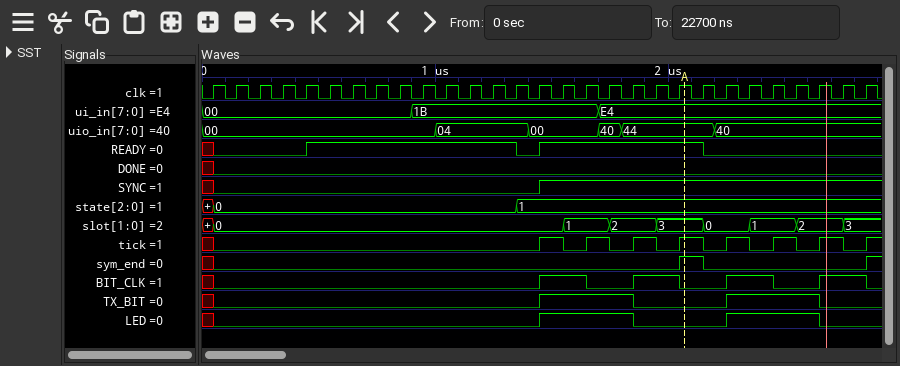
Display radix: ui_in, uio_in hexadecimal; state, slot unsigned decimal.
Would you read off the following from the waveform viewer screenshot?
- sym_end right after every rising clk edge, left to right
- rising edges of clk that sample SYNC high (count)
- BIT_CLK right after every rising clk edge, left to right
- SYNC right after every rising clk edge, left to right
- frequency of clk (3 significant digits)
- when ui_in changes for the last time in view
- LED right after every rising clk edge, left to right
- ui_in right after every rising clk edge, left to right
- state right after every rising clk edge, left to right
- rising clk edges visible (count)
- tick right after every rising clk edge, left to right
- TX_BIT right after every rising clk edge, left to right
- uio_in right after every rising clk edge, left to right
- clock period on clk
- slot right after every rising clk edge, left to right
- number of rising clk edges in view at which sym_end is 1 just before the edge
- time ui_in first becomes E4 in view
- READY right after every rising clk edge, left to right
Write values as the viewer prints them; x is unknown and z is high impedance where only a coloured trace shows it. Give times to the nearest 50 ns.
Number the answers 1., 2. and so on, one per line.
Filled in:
1. 0 0 0 0 0 0 0 0 0 0 0 0 0 0 0 0 0 0 0 0 1 0 0 0 0 0 0 0 1
2. 14
3. 0 0 0 0 0 0 0 0 0 0 0 0 0 0 1 1 0 0 1 1 0 0 1 1 0 0 1 1 0
4. 0 0 0 0 0 0 0 0 0 0 0 0 0 0 1 1 1 1 1 1 1 1 1 1 1 1 1 1 1
5. 10.0 MHz
6. 1700 ns
7. 0 0 0 0 0 0 0 0 0 0 0 0 0 0 1 1 1 1 0 0 0 0 1 1 1 1 0 0 0
8. 00, 00, 00, 00, 00, 00, 00, 00, 00, 1B, 1B, 1B, 1B, 1B, 1B, 1B, 1B, E4, E4, E4, E4, E4, E4, E4, E4, E4, E4, E4, E4
9. 0, 0, 0, 0, 0, 0, 0, 0, 0, 0, 0, 0, 0, 1, 1, 1, 1, 1, 1, 1, 1, 1, 1, 1, 1, 1, 1, 1, 1
10. 29
11. 0 0 0 0 0 0 0 0 0 0 0 0 0 0 1 0 1 0 1 0 1 0 1 0 1 0 1 0 1
12. 0 0 0 0 0 0 0 0 0 0 0 0 0 0 1 1 1 1 0 0 0 0 1 1 1 1 0 0 0
13. 00, 00, 00, 00, 00, 00, 00, 00, 00, 00, 04, 04, 04, 04, 00, 00, 00, 40, 44, 44, 44, 44, 40, 40, 40, 40, 40, 40, 40
14. 100 ns
15. 0, 0, 0, 0, 0, 0, 0, 0, 0, 0, 0, 0, 0, 0, 0, 1, 1, 2, 2, 3, 3, 0, 0, 1, 1, 2, 2, 3, 3
16. 1
17. 1700 ns
18. 0 0 0 0 1 1 1 1 1 1 1 1 1 0 1 1 1 1 1 1 1 0 0 0 0 0 0 0 0
